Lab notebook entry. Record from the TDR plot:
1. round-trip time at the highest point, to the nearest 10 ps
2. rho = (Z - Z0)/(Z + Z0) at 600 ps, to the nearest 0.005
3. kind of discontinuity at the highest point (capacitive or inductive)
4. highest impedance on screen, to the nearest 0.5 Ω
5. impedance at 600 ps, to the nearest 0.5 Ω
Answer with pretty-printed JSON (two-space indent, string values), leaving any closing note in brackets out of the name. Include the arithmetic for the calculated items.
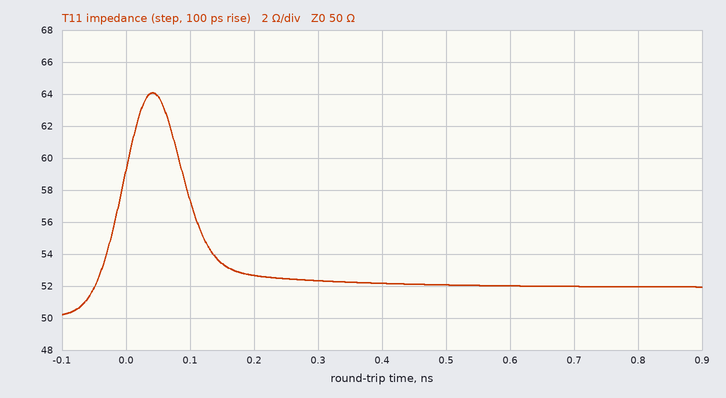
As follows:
{
  "round-trip time at the highest point, to the nearest 10 ps": "40 ps",
  "rho = (Z - Z0)/(Z + Z0) at 600 ps, to the nearest 0.005": "(52 − 50)/(52 + 50) ≈ +0.020",
  "kind of discontinuity at the highest point": "inductive",
  "highest impedance on screen, to the nearest 0.5 Ω": "64.0 Ω",
  "impedance at 600 ps, to the nearest 0.5 Ω": "52.0 Ω"
}
